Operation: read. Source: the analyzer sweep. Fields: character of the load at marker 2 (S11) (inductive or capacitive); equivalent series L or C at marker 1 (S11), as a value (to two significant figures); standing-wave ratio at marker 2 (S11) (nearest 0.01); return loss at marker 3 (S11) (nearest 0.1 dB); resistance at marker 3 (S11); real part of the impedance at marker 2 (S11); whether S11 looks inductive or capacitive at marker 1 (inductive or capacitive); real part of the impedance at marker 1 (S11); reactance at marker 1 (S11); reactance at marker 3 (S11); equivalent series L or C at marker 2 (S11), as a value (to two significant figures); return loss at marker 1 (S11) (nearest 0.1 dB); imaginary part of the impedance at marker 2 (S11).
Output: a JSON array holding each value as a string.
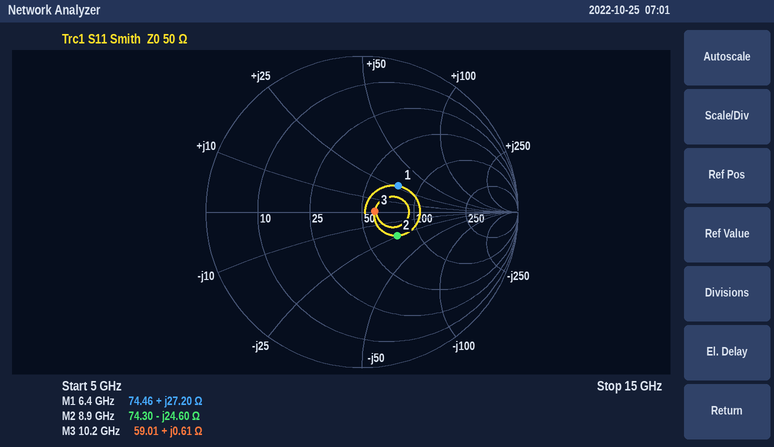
["capacitive", "680 pH", "1.75", "21.6 dB", "59.01 Ω", "74.30 Ω", "inductive", "74.46 Ω", "+27.20 Ω", "+0.61 Ω", "730 fF", "10.8 dB", "-24.60 Ω"]
